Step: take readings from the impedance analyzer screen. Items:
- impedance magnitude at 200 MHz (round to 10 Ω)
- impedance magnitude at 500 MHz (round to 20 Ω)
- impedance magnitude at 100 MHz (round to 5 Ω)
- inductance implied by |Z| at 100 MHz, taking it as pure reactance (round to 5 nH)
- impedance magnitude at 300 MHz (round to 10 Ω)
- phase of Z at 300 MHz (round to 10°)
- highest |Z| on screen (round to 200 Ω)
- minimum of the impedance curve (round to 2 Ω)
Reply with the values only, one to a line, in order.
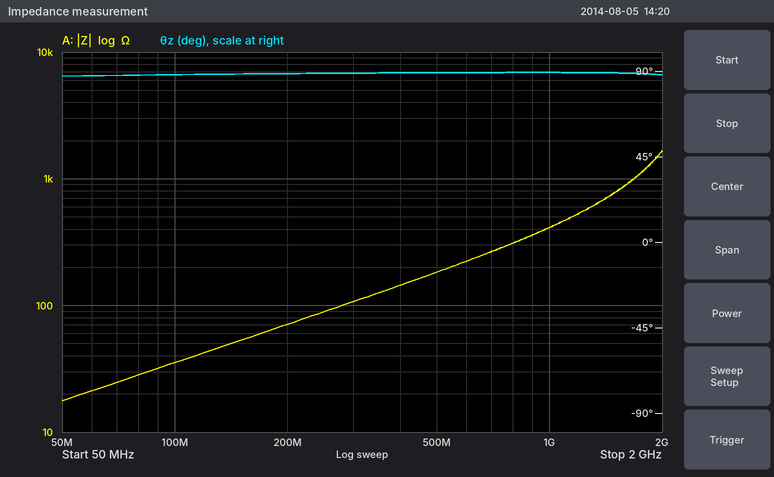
70 Ω
180 Ω
35 Ω
55 nH
110 Ω
90°
1.6 kΩ
18 Ω
